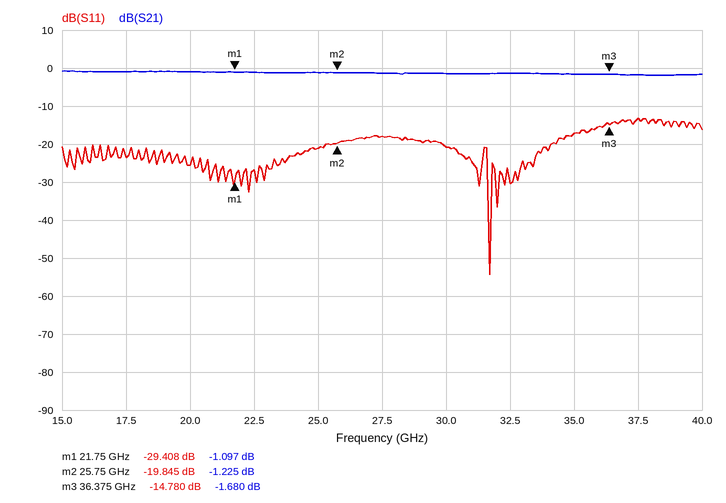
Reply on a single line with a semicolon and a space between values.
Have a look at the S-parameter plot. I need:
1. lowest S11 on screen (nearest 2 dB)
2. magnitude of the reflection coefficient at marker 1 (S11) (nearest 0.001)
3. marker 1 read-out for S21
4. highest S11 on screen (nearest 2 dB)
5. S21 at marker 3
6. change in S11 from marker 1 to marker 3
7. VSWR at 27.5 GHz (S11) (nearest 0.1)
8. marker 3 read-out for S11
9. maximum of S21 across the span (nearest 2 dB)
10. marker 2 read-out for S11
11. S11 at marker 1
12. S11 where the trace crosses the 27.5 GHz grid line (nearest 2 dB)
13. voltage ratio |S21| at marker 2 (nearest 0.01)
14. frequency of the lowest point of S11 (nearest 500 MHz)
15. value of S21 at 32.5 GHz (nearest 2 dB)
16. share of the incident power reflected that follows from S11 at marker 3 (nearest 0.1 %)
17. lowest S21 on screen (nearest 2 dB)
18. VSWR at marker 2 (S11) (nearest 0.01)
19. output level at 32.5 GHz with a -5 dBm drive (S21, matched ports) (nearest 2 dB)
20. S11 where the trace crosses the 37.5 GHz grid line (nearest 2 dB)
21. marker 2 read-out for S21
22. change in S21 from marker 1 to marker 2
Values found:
-54 dB; 0.034; -1.097 dB; -14 dB; -1.680 dB; 14.628 dB; 1.3; -14.780 dB; 0 dB; -19.845 dB; -29.408 dB; -18 dB; 0.87; 31.5 GHz; -2 dB; 3.3 %; -2 dB; 1.23; -6 dBm; -14 dB; -1.225 dB; -0.128 dB
